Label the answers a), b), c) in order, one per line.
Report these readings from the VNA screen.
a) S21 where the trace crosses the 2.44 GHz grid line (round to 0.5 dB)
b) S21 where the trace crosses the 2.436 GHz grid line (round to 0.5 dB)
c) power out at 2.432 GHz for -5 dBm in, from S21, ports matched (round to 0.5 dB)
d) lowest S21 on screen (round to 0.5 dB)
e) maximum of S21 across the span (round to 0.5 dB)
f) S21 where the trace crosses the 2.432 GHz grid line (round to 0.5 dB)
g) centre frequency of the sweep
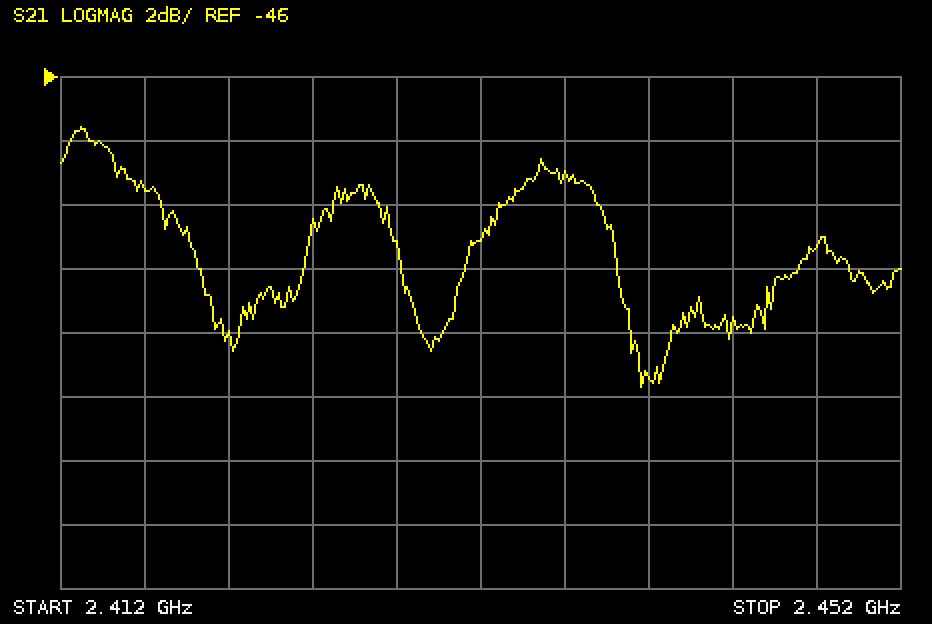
a) -55.5 dB
b) -49.0 dB
c) -56.0 dBm
d) -55.5 dB
e) -47.5 dB
f) -51.0 dB
g) 2.432 GHz
